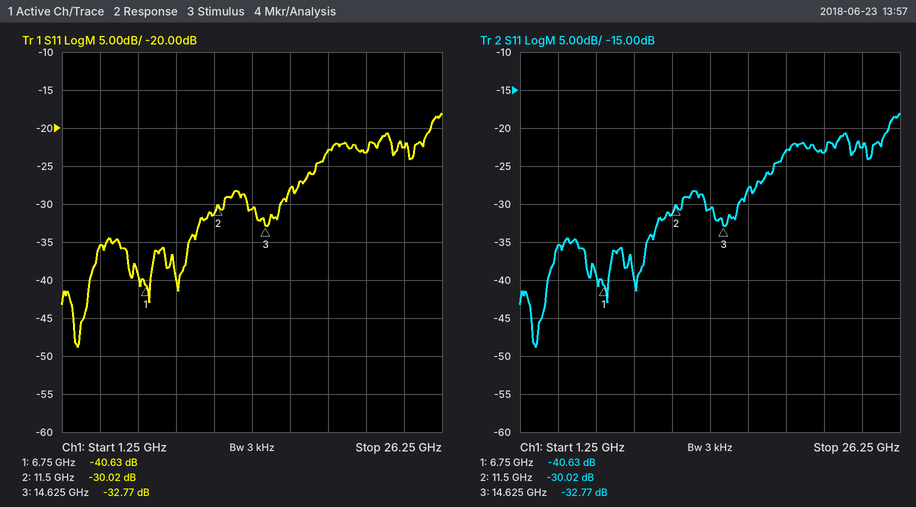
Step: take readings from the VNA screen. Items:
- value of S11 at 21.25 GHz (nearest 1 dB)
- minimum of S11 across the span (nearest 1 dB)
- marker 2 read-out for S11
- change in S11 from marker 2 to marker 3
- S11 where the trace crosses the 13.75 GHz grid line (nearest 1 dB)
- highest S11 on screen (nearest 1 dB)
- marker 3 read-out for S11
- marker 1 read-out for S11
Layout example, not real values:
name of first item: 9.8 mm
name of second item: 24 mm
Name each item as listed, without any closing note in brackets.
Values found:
value of S11 at 21.25 GHz: -23 dB
minimum of S11 across the span: -49 dB
marker 2 read-out for S11: -30.02 dB
change in S11 from marker 2 to marker 3: -2.75 dB
S11 where the trace crosses the 13.75 GHz grid line: -31 dB
highest S11 on screen: -18 dB
marker 3 read-out for S11: -32.77 dB
marker 1 read-out for S11: -40.63 dB
